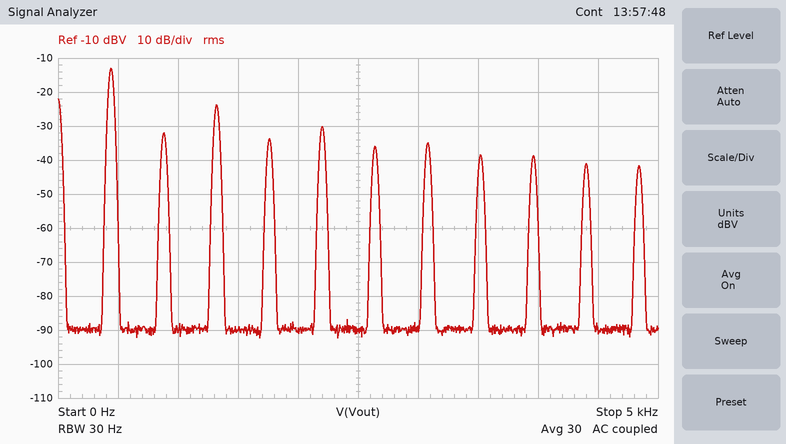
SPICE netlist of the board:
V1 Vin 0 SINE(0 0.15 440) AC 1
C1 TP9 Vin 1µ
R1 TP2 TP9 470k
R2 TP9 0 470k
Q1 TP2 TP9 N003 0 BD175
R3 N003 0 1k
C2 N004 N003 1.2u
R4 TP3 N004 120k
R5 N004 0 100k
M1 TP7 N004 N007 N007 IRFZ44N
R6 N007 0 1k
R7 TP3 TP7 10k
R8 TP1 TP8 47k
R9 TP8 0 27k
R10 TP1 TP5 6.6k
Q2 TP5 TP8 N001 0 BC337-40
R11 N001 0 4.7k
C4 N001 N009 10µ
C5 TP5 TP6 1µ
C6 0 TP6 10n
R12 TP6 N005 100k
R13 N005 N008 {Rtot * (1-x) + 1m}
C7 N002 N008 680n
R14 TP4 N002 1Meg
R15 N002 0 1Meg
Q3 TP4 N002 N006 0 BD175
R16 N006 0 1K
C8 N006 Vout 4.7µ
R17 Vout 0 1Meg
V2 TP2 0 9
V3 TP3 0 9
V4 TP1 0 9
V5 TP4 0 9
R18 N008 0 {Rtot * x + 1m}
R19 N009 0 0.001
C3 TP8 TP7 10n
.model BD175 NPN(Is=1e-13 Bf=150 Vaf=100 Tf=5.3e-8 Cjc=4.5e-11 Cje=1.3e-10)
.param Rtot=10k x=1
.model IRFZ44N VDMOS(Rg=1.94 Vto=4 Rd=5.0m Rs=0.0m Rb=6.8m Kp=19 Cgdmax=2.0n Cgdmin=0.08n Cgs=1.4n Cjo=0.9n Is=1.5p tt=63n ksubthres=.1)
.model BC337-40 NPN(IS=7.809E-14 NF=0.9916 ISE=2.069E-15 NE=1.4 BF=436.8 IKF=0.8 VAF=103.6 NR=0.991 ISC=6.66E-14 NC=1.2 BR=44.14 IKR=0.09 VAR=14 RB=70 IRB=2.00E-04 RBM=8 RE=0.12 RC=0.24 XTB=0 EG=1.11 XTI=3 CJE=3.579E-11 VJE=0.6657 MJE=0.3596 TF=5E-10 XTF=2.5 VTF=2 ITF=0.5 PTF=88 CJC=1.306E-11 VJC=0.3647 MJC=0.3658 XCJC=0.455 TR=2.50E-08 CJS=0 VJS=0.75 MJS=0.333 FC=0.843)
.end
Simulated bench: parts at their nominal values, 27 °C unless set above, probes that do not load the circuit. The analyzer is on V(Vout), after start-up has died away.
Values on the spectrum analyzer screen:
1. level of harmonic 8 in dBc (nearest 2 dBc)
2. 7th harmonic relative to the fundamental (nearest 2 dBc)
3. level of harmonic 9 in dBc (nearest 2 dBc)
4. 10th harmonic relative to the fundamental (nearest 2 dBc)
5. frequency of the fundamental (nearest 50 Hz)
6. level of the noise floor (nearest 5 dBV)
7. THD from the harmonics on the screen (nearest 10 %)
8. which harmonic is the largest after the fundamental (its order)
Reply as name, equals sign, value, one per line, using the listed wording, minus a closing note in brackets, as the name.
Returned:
level of harmonic 8 in dBc = -26 dBc
7th harmonic relative to the fundamental = -22 dBc
level of harmonic 9 in dBc = -26 dBc
10th harmonic relative to the fundamental = -28 dBc
frequency of the fundamental = 450 Hz
level of the noise floor = -90 dBV
THD from the harmonics on the screen = 40 %
which harmonic is the largest after the fundamental = 3
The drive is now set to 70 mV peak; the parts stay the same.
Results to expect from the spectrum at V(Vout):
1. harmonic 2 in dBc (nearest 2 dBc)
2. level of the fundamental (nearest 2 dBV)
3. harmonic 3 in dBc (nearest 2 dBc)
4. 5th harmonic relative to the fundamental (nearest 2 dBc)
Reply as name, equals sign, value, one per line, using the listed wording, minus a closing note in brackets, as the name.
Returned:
harmonic 2 in dBc = -16 dBc
level of the fundamental = -14 dBV
harmonic 3 in dBc = -12 dBc
5th harmonic relative to the fundamental = -20 dBc
